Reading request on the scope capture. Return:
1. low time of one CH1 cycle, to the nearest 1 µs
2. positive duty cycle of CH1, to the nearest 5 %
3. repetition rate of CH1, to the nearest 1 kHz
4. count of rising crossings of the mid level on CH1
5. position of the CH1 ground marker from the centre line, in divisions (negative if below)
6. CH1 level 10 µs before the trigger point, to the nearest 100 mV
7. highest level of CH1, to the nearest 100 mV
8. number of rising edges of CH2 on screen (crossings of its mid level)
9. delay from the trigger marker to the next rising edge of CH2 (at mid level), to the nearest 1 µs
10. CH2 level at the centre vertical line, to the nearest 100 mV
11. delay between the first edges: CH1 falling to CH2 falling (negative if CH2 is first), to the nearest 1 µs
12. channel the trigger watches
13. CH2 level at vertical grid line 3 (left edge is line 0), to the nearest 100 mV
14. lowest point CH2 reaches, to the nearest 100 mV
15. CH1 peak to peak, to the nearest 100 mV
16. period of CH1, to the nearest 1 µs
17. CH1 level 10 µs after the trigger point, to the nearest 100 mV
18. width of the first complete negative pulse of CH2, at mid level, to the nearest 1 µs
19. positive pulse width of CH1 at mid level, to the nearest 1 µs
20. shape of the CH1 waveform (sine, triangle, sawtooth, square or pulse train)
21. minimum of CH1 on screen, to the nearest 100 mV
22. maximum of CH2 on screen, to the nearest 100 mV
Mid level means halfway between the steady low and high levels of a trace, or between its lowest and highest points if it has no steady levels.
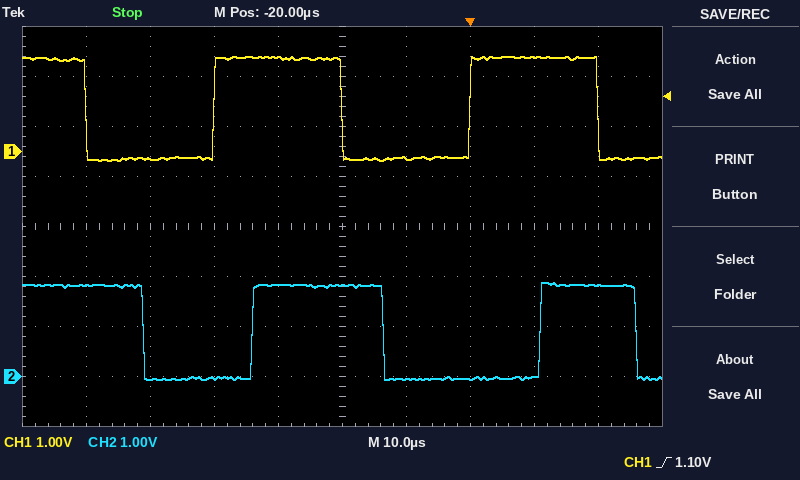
20 µs
50 %
25 kHz
2
+1.5 div
-100 mV
1.9 V
2
11 µs
1.8 V
+9 µs
CH1
0.0 V
-100 mV
2.1 V
40 µs
1.9 V
17 µs
20 µs
square
-200 mV
1.9 V
